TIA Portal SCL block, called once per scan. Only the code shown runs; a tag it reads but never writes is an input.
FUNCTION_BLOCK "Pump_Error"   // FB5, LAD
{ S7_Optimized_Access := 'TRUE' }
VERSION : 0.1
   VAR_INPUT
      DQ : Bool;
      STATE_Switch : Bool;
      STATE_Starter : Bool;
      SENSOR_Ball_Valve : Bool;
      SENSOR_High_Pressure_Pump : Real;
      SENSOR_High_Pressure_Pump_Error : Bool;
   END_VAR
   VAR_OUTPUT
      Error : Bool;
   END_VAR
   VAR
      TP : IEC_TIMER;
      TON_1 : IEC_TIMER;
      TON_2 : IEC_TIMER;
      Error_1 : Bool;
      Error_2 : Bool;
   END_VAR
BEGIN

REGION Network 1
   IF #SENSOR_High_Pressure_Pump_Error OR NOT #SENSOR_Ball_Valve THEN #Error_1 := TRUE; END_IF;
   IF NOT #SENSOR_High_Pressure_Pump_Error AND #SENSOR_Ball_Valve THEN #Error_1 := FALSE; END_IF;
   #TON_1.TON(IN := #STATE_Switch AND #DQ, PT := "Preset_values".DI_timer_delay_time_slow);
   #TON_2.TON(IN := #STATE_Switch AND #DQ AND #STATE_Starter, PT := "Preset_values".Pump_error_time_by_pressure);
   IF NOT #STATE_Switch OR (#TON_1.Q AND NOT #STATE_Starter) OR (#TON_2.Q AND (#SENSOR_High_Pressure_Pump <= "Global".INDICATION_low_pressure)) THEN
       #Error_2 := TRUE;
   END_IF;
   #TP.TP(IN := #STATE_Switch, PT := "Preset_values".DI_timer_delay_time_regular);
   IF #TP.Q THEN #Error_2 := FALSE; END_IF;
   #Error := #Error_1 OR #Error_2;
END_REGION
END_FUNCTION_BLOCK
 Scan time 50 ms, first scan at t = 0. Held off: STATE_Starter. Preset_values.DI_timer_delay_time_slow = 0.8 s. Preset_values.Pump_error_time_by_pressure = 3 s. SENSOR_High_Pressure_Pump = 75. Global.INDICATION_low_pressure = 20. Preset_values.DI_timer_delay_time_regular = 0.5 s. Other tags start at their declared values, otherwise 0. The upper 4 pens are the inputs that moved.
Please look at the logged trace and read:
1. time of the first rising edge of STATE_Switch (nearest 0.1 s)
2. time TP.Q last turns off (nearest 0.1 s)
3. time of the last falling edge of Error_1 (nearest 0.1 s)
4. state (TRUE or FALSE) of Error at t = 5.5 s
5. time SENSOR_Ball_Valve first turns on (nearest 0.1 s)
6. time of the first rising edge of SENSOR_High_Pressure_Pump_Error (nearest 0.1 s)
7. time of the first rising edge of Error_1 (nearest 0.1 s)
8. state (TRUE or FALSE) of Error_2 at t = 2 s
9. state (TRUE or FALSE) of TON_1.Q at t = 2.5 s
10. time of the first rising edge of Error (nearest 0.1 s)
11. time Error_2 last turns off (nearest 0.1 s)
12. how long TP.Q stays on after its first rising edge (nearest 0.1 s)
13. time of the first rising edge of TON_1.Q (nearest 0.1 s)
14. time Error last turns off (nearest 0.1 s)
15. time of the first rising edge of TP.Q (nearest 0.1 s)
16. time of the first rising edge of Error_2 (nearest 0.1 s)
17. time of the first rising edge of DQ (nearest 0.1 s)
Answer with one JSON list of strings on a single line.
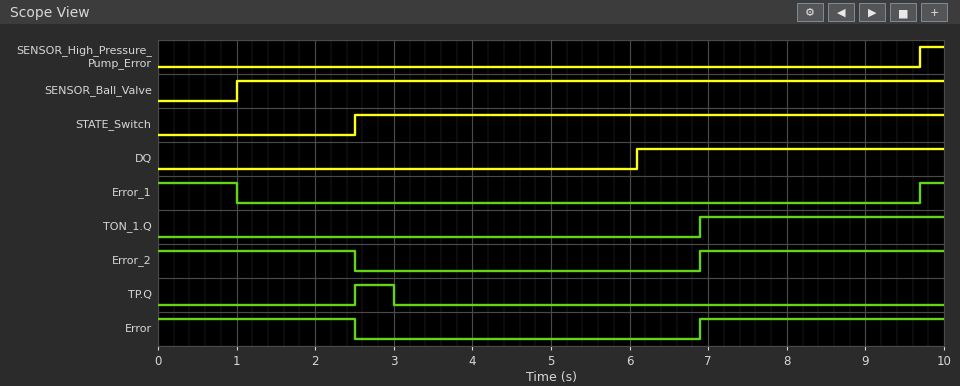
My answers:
["2.5 s", "3.0 s", "1.0 s", "FALSE", "1.0 s", "9.7 s", "9.7 s", "TRUE", "FALSE", "6.9 s", "2.5 s", "0.5 s", "6.9 s", "2.5 s", "2.5 s", "6.9 s", "6.1 s"]
